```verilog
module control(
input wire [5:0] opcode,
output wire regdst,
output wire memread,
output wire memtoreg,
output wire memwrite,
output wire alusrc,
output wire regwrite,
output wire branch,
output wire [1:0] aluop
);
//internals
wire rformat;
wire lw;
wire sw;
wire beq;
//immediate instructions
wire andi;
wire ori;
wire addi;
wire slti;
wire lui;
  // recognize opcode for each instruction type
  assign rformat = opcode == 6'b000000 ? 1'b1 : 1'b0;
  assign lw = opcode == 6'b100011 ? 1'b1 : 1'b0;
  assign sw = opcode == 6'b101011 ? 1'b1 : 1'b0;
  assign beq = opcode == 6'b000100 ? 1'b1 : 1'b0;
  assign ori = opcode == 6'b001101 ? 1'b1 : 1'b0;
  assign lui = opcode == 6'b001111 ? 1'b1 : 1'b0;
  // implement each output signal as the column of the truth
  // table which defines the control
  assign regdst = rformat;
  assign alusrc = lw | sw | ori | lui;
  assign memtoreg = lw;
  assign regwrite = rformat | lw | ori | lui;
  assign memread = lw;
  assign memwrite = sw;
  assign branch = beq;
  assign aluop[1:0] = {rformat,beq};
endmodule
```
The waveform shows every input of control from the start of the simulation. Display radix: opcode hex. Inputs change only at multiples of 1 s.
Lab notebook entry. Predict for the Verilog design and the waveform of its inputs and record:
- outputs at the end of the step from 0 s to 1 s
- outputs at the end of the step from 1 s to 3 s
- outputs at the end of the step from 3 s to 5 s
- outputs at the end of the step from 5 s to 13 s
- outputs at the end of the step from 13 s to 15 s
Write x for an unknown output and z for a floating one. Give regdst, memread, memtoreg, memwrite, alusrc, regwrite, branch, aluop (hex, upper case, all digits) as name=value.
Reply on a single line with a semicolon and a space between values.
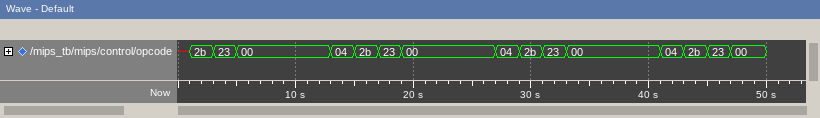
regdst=x, memread=x, memtoreg=x, memwrite=x, alusrc=x, regwrite=x, branch=x, aluop=x; regdst=0, memread=0, memtoreg=0, memwrite=1, alusrc=1, regwrite=0, branch=0, aluop=0; regdst=0, memread=1, memtoreg=1, memwrite=0, alusrc=1, regwrite=1, branch=0, aluop=0; regdst=1, memread=0, memtoreg=0, memwrite=0, alusrc=0, regwrite=1, branch=0, aluop=2; regdst=0, memread=0, memtoreg=0, memwrite=0, alusrc=0, regwrite=0, branch=1, aluop=1
